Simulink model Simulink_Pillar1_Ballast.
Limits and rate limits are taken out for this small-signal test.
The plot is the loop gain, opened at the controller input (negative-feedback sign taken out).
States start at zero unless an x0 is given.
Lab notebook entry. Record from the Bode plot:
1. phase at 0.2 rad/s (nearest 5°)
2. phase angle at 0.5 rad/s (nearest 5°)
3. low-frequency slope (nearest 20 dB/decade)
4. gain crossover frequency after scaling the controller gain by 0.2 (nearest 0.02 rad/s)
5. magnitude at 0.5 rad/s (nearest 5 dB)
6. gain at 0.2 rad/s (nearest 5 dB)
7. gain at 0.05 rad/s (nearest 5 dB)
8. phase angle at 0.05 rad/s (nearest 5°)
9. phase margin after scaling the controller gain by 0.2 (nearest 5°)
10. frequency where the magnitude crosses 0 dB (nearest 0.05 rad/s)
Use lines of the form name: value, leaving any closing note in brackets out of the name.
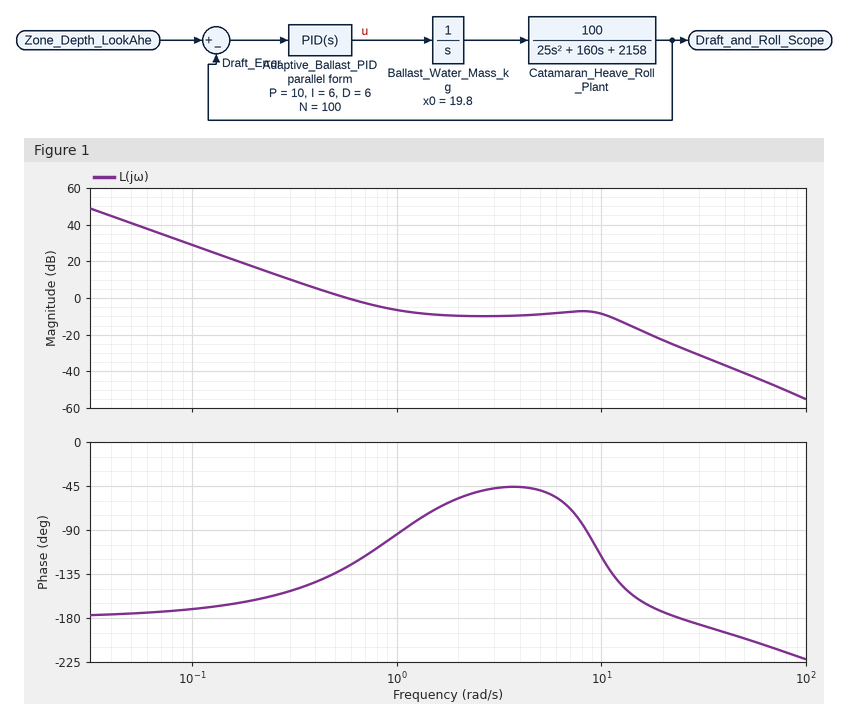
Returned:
phase at 0.2 rad/s: -160°
phase angle at 0.5 rad/s: -135°
low-frequency slope: -40 dB/decade
gain crossover frequency after scaling the controller gain by 0.2: 0.24 rad/s
magnitude at 0.5 rad/s: 0 dB
gain at 0.2 rad/s: 15 dB
gain at 0.05 rad/s: 40 dB
phase angle at 0.05 rad/s: -175°
phase margin after scaling the controller gain by 0.2: 20°
frequency where the magnitude crosses 0 dB: 0.55 rad/s
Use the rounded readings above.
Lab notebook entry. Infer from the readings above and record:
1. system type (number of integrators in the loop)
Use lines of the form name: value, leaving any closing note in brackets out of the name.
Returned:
system type: 2
